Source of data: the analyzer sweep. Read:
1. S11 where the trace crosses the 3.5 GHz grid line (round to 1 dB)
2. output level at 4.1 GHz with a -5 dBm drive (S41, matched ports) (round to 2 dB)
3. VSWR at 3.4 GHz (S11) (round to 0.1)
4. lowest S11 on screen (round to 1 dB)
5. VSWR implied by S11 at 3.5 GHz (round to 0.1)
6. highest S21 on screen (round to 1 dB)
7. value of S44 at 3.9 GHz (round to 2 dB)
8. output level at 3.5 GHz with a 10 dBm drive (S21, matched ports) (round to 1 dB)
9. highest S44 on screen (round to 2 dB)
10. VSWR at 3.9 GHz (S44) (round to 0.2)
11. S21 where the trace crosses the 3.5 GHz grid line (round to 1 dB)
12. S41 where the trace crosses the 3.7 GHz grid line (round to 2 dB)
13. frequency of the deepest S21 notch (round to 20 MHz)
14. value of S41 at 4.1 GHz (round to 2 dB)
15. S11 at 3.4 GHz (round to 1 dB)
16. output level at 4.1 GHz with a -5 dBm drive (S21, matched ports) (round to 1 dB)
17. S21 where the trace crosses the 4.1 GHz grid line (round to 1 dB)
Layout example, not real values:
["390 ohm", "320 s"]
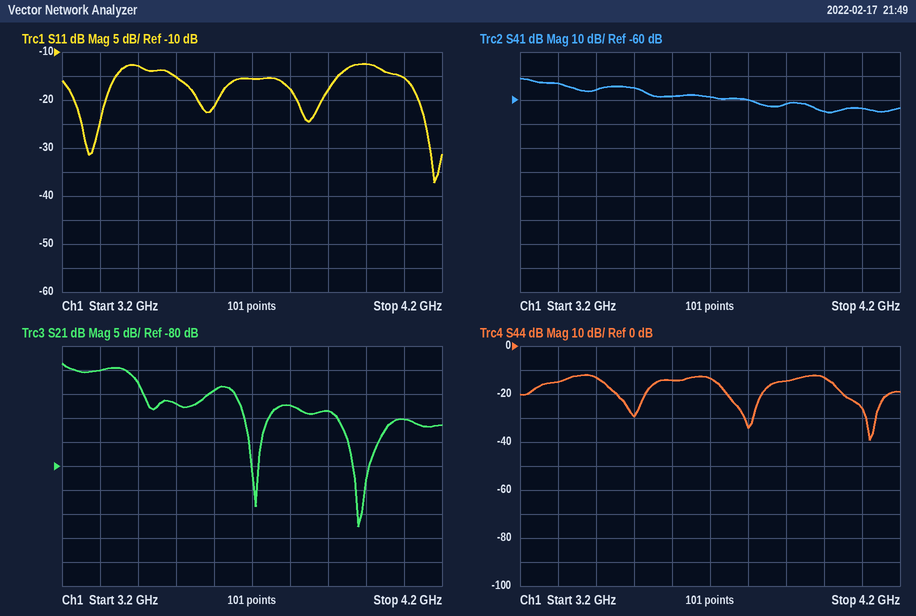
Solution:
["-15 dB", "-68 dBm", "1.6", "-37 dB", "1.4", "-59 dB", "-14 dB", "-57 dBm", "-12 dB", "1.4", "-67 dB", "-58 dB", "3.98 GHz", "-64 dB", "-13 dB", "-75 dBm", "-70 dB"]
